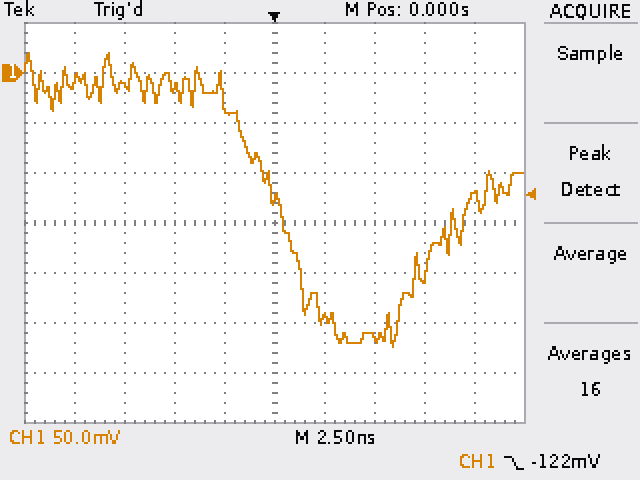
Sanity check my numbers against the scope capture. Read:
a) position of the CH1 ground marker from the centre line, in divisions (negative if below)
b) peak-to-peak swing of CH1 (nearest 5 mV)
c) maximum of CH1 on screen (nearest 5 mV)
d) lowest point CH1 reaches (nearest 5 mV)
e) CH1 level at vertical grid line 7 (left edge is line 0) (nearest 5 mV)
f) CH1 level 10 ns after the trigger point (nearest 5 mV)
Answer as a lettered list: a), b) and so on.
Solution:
a) +3.0 div
b) 295 mV
c) 20 mV
d) -275 mV
e) -265 mV
f) -125 mV
